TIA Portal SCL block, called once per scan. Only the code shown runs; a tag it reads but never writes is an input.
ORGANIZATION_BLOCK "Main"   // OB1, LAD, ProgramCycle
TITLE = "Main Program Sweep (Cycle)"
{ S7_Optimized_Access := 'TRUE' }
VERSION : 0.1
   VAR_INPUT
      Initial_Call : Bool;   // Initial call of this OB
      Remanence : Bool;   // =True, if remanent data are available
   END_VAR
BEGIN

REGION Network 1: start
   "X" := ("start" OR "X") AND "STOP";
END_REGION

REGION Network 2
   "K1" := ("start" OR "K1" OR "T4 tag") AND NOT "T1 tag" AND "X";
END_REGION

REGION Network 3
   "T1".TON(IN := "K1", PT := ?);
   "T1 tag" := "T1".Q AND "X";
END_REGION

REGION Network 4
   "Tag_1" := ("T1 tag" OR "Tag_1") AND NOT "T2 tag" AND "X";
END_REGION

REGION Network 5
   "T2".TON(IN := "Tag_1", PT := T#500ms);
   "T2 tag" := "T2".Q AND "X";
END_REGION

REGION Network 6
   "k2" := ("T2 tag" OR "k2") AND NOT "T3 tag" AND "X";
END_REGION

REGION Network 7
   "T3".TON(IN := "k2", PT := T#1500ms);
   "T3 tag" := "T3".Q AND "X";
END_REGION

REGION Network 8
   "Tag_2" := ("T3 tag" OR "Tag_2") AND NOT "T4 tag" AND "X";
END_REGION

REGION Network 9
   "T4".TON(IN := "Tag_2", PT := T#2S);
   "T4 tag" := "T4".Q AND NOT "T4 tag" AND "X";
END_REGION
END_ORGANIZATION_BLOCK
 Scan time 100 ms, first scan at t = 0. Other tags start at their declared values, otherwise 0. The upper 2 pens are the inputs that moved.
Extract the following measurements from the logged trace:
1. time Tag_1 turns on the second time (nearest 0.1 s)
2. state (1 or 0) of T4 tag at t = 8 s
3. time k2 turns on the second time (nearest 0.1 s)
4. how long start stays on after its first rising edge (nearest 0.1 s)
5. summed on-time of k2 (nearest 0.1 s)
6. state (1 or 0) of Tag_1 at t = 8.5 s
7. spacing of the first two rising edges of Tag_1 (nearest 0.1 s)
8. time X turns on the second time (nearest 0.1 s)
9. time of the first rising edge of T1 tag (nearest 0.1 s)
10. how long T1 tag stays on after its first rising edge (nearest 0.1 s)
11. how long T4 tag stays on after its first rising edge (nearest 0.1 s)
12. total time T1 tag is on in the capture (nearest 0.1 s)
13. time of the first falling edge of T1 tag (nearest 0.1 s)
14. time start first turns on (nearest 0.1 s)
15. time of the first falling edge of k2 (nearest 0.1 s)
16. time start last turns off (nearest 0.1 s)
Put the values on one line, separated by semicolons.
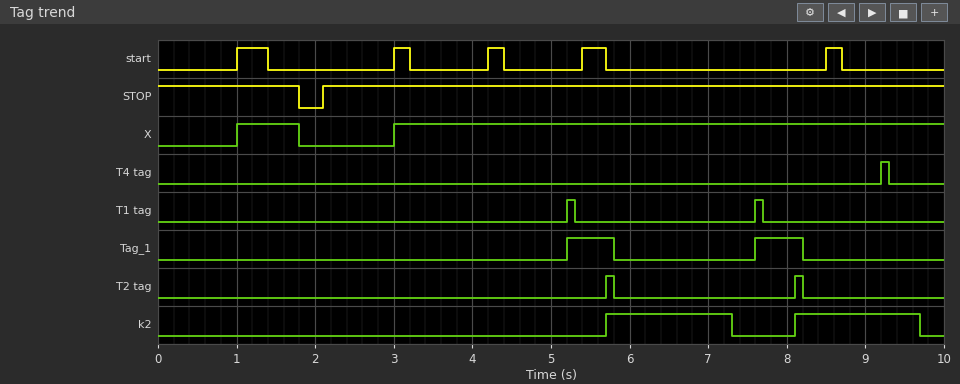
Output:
7.6 s; 0; 8.1 s; 0.4 s; 3.2 s; 0; 2.4 s; 3.0 s; 5.2 s; 0.1 s; 0.1 s; 0.2 s; 5.3 s; 1.0 s; 7.3 s; 8.7 s
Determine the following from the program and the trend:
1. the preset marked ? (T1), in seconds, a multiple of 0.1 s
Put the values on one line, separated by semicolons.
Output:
2.2 s
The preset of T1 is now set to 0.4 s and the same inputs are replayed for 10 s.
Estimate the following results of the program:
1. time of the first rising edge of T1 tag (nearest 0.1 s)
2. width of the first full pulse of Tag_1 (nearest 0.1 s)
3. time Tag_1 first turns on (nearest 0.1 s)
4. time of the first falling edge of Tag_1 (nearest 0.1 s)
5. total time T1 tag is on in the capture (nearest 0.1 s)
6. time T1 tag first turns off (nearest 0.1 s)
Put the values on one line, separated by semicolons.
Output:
1.4 s; 0.4 s; 1.4 s; 1.8 s; 0.6 s; 1.5 s
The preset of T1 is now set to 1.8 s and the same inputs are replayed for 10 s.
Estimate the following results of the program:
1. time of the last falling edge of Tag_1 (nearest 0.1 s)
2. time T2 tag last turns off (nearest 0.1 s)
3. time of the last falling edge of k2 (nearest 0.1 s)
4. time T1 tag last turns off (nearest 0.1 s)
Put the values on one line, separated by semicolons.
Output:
7.8 s; 7.8 s; 9.3 s; 7.3 s
